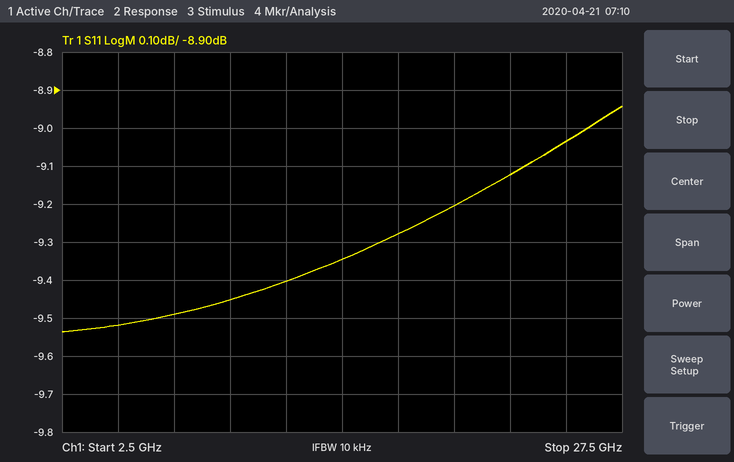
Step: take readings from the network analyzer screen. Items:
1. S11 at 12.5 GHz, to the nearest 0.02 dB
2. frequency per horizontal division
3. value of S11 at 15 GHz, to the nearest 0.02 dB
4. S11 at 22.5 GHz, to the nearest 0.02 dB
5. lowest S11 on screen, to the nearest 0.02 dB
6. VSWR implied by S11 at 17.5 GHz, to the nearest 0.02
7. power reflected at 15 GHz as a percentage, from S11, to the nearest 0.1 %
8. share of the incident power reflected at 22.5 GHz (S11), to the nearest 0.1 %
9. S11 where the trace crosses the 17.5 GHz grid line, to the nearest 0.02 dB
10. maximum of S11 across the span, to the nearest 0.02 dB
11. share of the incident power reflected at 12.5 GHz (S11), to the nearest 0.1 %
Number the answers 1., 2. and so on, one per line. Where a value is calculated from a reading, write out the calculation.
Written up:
1. -9.40 dB
2. 2.5 GHz
3. -9.34 dB
4. -9.12 dB
5. -9.54 dB
6. |Γ| = 10^(-9.28/20) = 0.3436; VSWR = (1 + 0.3436)/(1 − 0.3436) ≈ 2.05, so 2.04 to the nearest 0.02
7. 10^(-9.34/10) ≈ 11.6 %
8. 10^(-9.12/10) ≈ 12.2 %
9. -9.28 dB
10. -8.94 dB
11. 10^(-9.4/10) ≈ 11.5 %
